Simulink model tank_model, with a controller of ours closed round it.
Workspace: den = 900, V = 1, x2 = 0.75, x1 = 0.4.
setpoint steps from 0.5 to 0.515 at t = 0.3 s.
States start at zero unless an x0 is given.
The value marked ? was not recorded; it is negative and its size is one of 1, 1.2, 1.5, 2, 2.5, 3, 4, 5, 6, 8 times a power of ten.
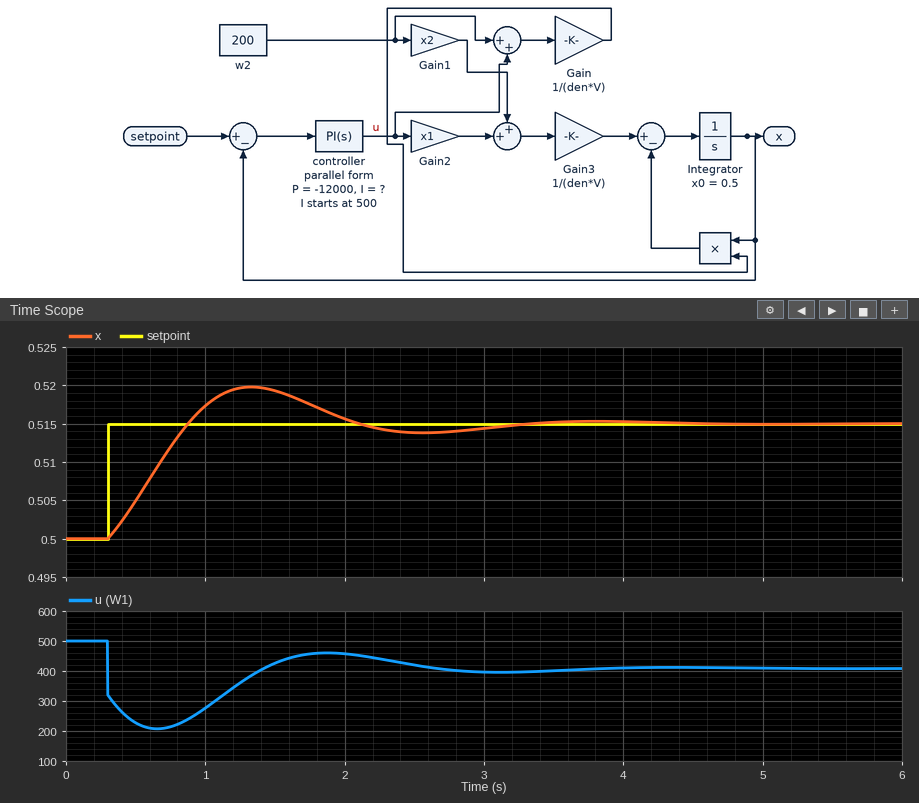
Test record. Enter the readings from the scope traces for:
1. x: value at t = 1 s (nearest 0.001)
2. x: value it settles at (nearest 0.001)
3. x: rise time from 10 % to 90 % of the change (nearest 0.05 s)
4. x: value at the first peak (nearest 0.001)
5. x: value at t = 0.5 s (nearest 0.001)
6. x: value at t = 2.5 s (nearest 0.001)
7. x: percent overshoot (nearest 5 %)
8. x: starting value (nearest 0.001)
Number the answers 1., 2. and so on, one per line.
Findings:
1. 0.517
2. 0.515
3. 0.45 s
4. 0.520
5. 0.505
6. 0.514
7. 30 %
8. 0.500
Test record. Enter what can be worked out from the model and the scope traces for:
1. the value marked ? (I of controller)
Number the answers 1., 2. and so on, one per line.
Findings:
1. -60000
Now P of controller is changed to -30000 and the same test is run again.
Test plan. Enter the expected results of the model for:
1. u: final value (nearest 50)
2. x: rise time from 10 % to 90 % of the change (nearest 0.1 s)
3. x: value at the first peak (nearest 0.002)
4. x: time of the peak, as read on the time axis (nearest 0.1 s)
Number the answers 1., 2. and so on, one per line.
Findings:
1. 400
2. 0.4 s
3. 0.516
4. 1.2 s
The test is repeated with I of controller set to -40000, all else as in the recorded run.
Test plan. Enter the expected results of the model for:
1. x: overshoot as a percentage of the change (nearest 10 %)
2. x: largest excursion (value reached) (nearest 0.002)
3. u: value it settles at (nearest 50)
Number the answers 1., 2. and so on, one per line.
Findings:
1. 20 %
2. 0.518
3. 400
